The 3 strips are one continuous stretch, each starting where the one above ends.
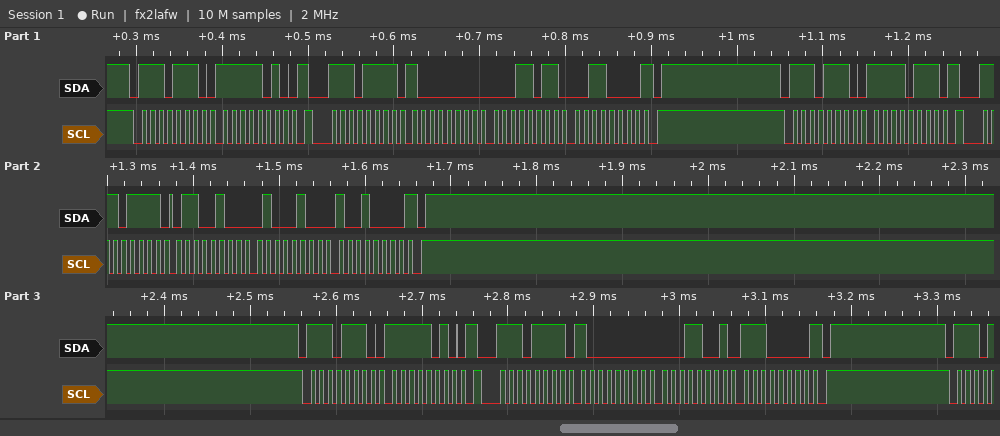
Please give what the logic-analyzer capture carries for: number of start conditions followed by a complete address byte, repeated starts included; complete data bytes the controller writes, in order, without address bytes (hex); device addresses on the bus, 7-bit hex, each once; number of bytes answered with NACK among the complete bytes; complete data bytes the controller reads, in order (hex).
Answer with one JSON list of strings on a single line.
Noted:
["6", "FA F7 FA", "0x77", "3", "80 1B 30 64 44 90 80 19 E0"]
